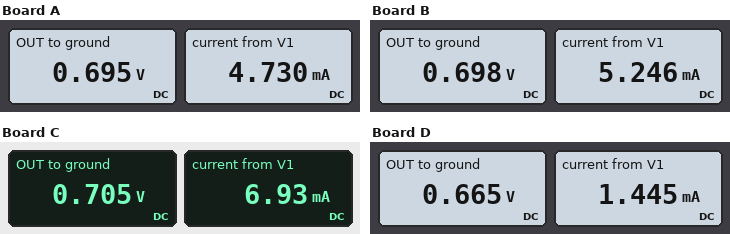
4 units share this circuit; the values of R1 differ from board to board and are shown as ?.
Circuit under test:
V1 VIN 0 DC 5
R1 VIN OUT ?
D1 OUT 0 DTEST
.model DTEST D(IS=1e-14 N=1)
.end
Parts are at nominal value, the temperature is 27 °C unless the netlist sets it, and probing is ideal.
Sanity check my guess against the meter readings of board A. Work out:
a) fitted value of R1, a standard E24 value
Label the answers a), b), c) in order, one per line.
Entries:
a) 910 Ω
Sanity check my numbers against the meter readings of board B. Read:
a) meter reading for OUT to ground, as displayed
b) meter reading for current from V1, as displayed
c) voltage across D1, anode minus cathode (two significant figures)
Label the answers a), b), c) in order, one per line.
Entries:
a) 0.698 V
b) 5.246 mA
c) 700 mV
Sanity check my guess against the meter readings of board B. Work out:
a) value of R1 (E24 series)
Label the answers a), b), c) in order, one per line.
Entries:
a) 820 Ω
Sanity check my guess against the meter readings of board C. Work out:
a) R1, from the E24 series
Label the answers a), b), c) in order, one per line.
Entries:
a) 620 Ω
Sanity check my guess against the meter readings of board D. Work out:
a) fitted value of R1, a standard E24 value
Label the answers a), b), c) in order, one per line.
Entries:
a) 3 kΩ
